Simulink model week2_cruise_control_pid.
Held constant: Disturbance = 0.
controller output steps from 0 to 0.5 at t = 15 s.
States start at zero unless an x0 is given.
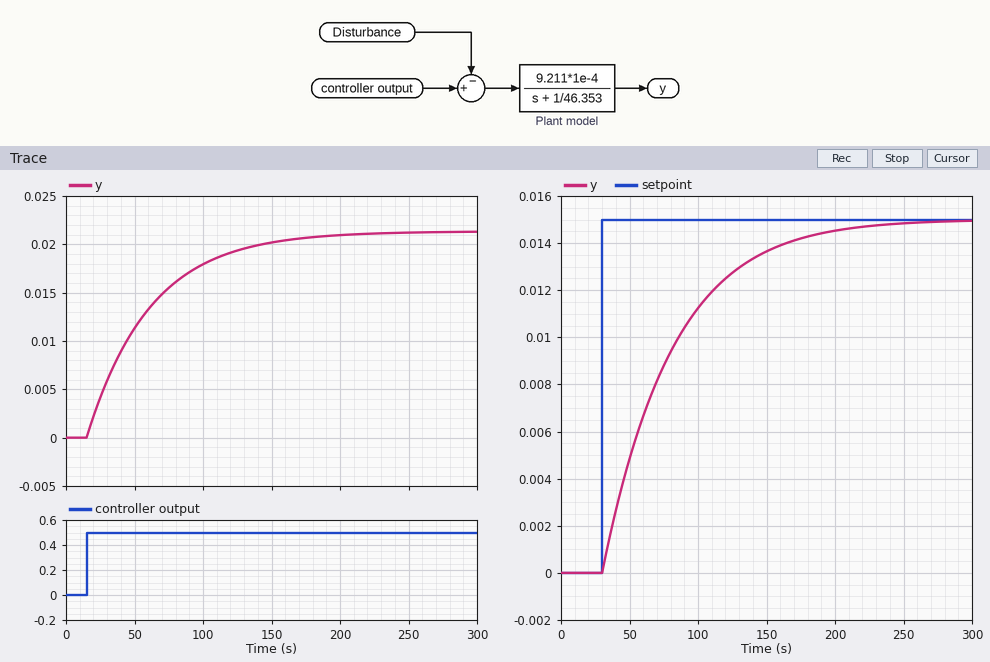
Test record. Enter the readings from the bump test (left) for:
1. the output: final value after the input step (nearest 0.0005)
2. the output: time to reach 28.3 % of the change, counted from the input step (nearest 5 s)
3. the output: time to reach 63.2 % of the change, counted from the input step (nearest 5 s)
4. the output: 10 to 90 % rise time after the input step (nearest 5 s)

0.0215
15 s
45 s
100 s
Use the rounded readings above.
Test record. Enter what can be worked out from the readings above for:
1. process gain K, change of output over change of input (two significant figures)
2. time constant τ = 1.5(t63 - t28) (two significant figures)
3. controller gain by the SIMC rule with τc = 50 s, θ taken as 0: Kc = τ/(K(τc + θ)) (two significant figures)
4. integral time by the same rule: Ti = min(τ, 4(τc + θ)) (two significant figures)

0.043
45 s
21
45 s
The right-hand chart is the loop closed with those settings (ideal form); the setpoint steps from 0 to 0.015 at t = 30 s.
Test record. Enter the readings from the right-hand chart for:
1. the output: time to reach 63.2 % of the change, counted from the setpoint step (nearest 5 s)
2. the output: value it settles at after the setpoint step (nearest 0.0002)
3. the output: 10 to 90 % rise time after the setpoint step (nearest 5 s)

50 s
0.0150
110 s
